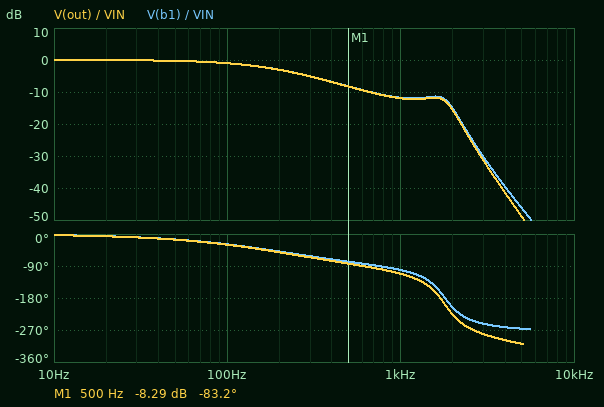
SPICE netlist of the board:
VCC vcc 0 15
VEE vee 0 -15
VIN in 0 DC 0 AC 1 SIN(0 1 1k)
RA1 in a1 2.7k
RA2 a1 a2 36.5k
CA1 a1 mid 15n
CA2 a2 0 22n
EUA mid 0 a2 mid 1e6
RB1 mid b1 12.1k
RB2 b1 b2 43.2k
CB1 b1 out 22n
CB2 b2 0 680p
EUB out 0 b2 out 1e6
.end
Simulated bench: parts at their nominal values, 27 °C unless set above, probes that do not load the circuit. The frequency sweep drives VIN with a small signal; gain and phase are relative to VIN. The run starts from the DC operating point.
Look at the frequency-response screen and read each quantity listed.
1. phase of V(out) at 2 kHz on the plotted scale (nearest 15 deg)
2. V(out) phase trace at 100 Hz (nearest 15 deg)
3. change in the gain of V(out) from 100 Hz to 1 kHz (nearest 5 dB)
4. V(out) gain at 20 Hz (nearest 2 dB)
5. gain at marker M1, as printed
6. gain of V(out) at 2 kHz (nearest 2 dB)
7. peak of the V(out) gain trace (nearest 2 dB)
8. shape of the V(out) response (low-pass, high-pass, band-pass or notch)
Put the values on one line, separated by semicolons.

-225 deg; -30 deg; -10 dB; 0 dB; -8.29 dB; -16 dB; 0 dB; low-pass
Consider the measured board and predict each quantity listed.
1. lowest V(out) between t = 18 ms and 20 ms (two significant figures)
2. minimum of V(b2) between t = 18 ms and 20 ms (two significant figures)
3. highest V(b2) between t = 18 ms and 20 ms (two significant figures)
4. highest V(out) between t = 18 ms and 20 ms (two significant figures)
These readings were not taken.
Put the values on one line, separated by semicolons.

-250 mV; -250 mV; 250 mV; 250 mV
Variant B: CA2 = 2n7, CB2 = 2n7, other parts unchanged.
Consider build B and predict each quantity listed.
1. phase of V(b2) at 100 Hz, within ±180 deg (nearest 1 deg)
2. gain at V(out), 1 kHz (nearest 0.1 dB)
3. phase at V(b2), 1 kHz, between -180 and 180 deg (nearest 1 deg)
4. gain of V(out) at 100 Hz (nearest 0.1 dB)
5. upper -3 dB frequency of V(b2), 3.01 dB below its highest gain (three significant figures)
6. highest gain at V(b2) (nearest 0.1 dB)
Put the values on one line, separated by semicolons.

-9 deg; -0.3 dB; -142 deg; 0.1 dB; 1.05 kHz; 2.0 dB
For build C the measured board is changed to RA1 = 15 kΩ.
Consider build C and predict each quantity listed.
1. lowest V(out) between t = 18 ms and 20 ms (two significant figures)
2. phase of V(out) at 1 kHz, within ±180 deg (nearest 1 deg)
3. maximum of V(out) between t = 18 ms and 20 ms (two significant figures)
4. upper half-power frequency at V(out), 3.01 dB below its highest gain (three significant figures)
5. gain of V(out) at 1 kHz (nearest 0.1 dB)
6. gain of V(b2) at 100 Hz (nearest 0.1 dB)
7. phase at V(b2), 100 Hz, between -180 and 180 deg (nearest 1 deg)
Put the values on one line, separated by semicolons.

-150 mV; -150 deg; 150 mV; 165 Hz; -16.7 dB; -1.3 dB; -39 deg
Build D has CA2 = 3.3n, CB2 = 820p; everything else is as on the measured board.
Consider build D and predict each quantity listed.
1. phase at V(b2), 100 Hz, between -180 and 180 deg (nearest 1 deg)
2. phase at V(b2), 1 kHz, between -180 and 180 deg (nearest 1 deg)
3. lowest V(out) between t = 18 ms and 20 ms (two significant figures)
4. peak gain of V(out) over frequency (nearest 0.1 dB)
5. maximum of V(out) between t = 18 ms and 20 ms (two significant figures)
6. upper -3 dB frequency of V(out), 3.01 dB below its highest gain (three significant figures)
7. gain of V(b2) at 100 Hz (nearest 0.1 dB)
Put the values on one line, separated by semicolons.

-6 deg; -70 deg; -1.3 V; 4.2 dB; 1.3 V; 1.82 kHz; 0 dB
